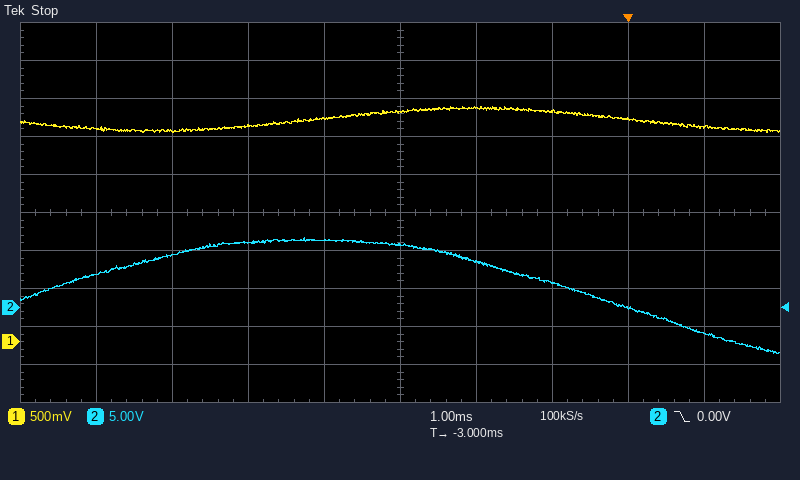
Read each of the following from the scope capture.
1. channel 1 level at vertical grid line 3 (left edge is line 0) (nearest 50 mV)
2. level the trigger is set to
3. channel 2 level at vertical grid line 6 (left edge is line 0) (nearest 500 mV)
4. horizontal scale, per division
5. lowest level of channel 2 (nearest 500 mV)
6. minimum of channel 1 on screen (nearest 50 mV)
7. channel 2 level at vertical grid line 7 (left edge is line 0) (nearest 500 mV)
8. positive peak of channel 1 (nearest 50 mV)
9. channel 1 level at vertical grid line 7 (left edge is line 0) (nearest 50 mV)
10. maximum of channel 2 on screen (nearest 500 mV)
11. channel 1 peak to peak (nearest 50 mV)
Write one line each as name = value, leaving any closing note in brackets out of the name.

channel 1 level at vertical grid line 3 (left edge is line 0) = 2.85 V
level the trigger is set to = 0.00 V
channel 2 level at vertical grid line 6 (left edge is line 0) = 6.0 V
horizontal scale, per division = 1 ms
lowest level of channel 2 = -6.0 V
minimum of channel 1 on screen = 2.75 V
channel 2 level at vertical grid line 7 (left edge is line 0) = 3.5 V
positive peak of channel 1 = 3.10 V
channel 1 level at vertical grid line 7 (left edge is line 0) = 3.05 V
maximum of channel 2 on screen = 9.0 V
channel 1 peak to peak = 350 mV
